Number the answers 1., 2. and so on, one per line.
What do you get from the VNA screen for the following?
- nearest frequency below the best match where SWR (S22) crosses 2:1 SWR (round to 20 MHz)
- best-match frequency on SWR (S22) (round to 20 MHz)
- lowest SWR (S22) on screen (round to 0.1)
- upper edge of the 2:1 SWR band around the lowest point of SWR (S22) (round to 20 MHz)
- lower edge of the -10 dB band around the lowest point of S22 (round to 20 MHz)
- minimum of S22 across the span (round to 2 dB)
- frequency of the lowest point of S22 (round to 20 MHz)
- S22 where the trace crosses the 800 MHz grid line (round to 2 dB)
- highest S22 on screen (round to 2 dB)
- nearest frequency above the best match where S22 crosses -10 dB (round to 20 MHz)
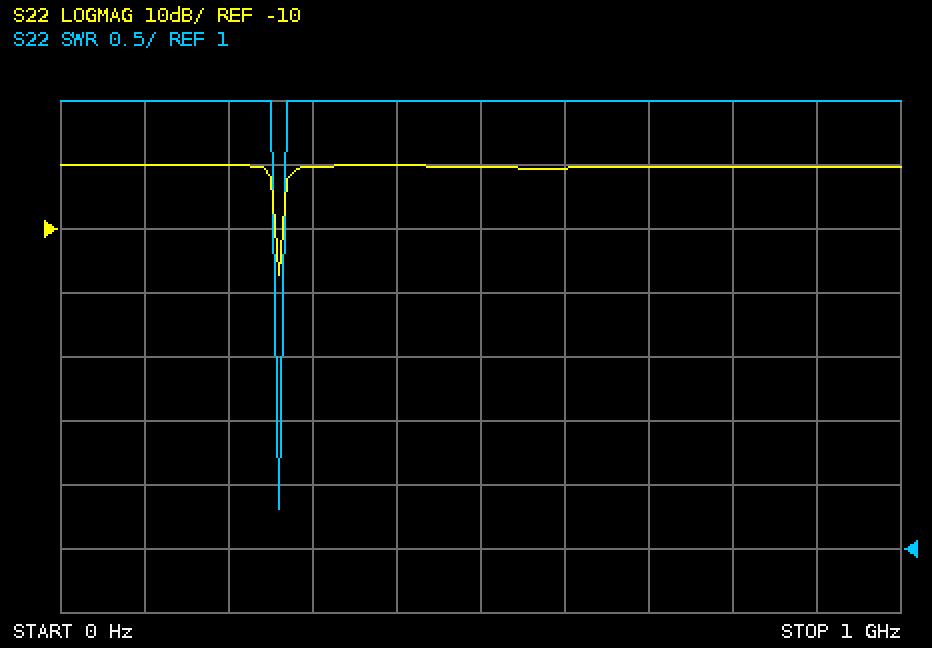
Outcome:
1. 260 MHz
2. 260 MHz
3. 1.3
4. 260 MHz
5. 260 MHz
6. -18 dB
7. 260 MHz
8. 0 dB
9. 0 dB
10. 260 MHz
